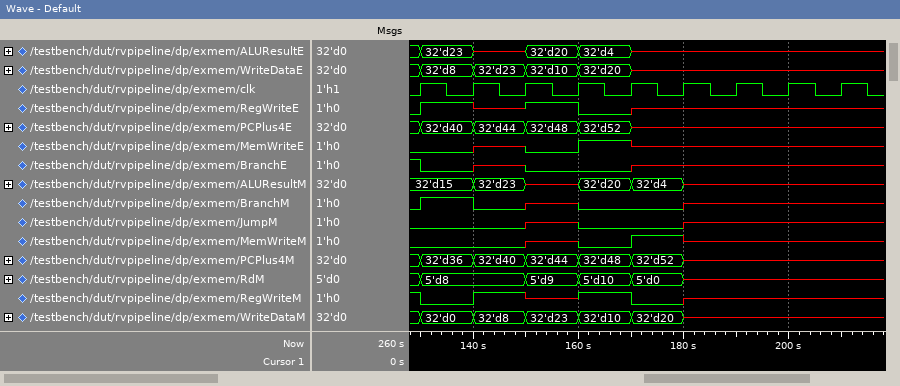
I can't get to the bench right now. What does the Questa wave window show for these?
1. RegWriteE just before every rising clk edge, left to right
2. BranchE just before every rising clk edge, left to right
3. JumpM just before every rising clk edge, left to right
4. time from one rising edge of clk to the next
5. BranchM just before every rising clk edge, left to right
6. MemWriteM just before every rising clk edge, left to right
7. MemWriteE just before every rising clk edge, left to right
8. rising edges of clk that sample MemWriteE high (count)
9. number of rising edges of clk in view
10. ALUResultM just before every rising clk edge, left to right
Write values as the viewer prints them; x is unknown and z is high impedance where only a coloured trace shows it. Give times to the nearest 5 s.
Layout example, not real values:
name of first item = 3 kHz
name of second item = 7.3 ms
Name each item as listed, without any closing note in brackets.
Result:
RegWriteE just before every rising clk edge, left to right = 0 1 x 1 0 x x x x
BranchE just before every rising clk edge, left to right = 1 0 x 0 0 x x x x
JumpM just before every rising clk edge, left to right = 0 0 0 x 0 0 x x x
time from one rising edge of clk to the next = 10 s
BranchM just before every rising clk edge, left to right = 0 1 0 x 0 0 x x x
MemWriteM just before every rising clk edge, left to right = 0 0 0 x 0 1 x x x
MemWriteE just before every rising clk edge, left to right = 0 0 x 0 1 x x x x
rising edges of clk that sample MemWriteE high = 1
number of rising edges of clk in view = 9
ALUResultM just before every rising clk edge, left to right = 32'd15, 32'd15, 32'd23, x, 32'd20, 32'd4, x, x, x
